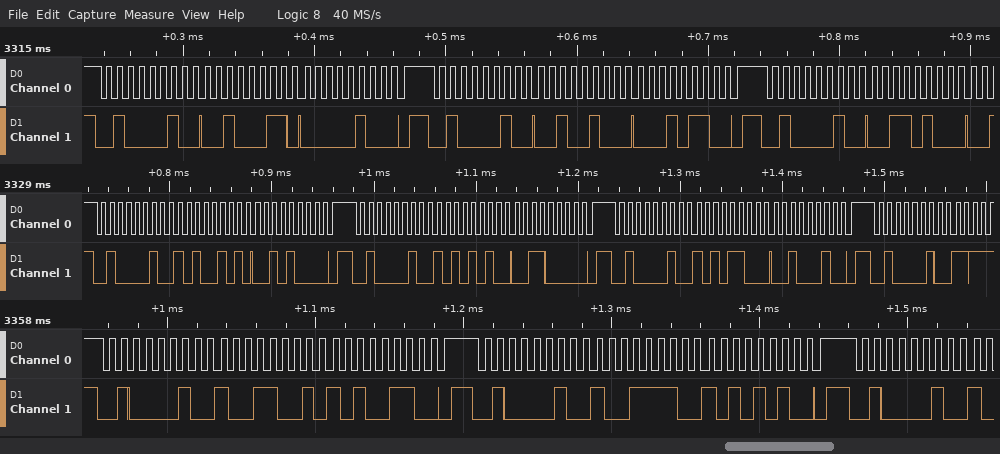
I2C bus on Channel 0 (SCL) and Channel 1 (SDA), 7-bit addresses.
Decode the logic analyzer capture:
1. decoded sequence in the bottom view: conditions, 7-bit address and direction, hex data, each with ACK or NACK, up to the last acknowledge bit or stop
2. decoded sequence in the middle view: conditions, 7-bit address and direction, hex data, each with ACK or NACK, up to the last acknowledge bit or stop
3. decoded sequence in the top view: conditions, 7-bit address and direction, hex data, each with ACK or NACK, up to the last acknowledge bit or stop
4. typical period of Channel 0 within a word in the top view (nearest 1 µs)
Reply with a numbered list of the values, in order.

1. start, address 21 write ACK, 99 ACK, A6 ACK, stop, start, address 21 write ACK, 9E ACK, AA ACK, stop, start, address 21 write ACK
2. start, address 21 write ACK, A5 ACK, 28 ACK, stop, start, address 21 write ACK, AA ACK, 30 ACK, stop, start, address 21 write ACK, AC ACK, 22 ACK, stop, start, address 21 write ACK
3. start, address 21 write ACK, 23 ACK, 04 ACK, stop, start, address 21 write ACK, 24 ACK, 16 ACK, stop, start, address 21 write ACK, 34 ACK
4. 8 µs
